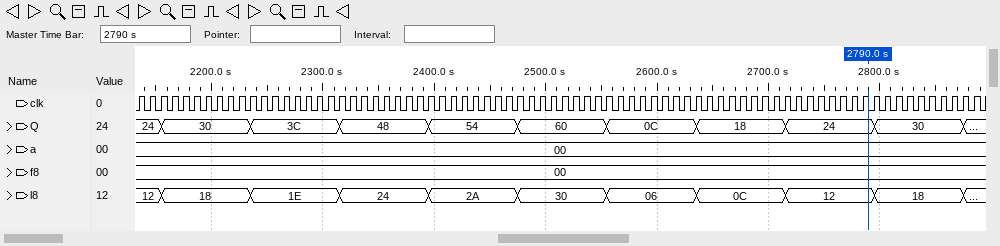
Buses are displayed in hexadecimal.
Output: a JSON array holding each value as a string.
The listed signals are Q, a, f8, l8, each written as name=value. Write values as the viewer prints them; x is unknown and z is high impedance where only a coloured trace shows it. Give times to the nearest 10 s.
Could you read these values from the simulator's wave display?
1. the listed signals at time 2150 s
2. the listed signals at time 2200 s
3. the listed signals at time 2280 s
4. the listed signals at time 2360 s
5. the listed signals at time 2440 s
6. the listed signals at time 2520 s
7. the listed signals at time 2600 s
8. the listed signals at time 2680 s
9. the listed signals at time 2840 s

["Q=24, a=00, f8=00, l8=12", "Q=30, a=00, f8=00, l8=18", "Q=3C, a=00, f8=00, l8=1E", "Q=48, a=00, f8=00, l8=24", "Q=54, a=00, f8=00, l8=2A", "Q=60, a=00, f8=00, l8=30", "Q=0C, a=00, f8=00, l8=06", "Q=18, a=00, f8=00, l8=0C", "Q=30, a=00, f8=00, l8=18"]
